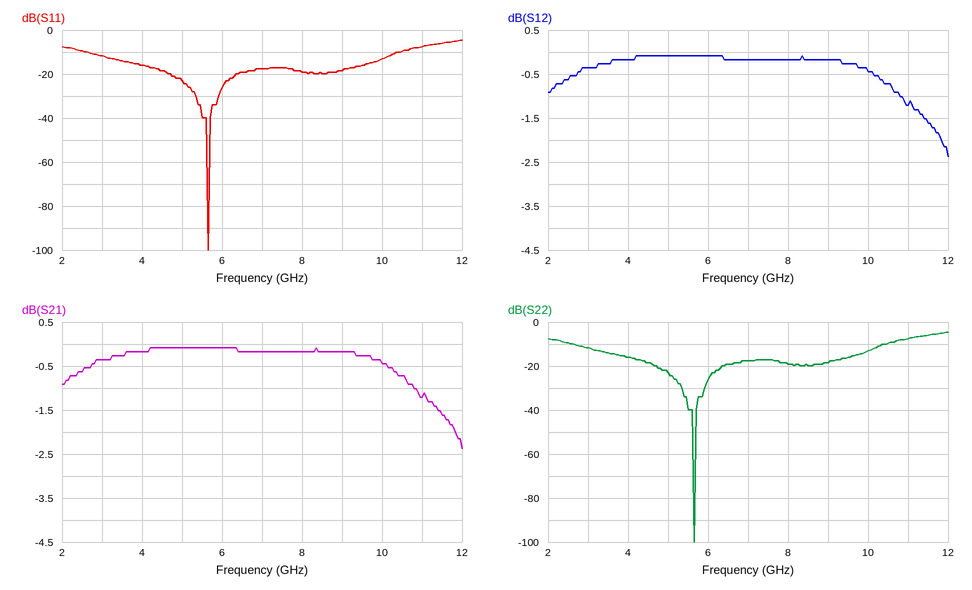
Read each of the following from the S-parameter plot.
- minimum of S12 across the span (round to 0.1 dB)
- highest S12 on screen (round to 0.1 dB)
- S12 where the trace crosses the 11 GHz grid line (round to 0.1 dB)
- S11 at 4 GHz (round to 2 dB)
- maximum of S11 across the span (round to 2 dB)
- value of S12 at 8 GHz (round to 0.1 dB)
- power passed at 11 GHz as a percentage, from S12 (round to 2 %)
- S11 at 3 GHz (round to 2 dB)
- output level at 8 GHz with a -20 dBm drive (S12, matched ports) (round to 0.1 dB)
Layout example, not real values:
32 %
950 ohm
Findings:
-2.4 dB
-0.1 dB
-1.2 dB
-16 dB
-4 dB
-0.2 dB
76 %
-12 dB
-20.2 dBm
